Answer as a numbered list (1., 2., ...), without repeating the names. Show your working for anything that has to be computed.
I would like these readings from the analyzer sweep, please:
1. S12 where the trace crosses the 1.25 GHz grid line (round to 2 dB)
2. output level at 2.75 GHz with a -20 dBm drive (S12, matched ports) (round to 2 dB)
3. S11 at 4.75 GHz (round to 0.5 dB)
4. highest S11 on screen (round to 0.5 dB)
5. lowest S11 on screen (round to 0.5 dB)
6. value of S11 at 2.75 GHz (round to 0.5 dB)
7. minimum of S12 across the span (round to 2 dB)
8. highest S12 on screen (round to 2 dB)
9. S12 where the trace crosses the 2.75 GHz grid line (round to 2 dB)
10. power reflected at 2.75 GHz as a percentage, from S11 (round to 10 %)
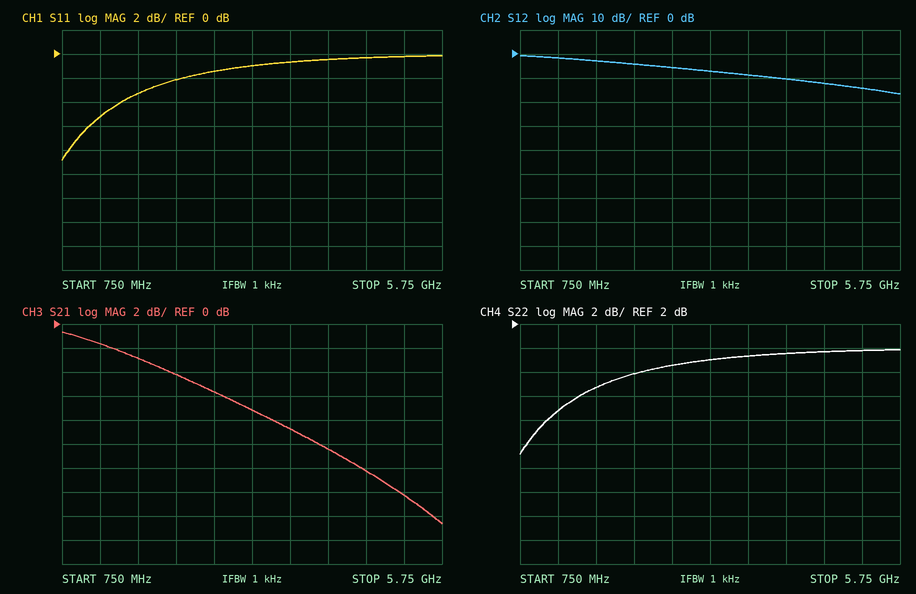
1. -2 dB
2. -20 dBm + (-6 dB) = -26 dBm
3. -0.5 dB
4. 0.0 dB
5. -9.0 dB
6. -1.5 dB
7. -16 dB
8. 0 dB
9. -6 dB
10. 10^(-1.5/10) ≈ 70.8 %, so 70 % to the nearest 10 %
